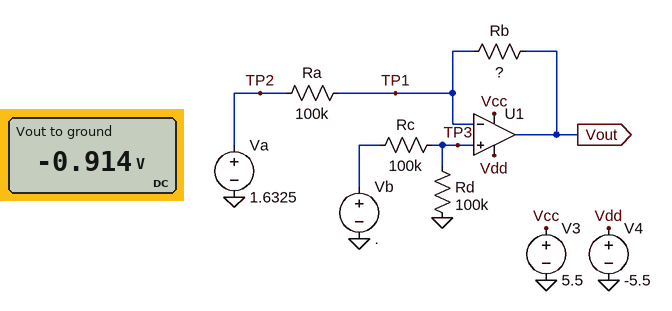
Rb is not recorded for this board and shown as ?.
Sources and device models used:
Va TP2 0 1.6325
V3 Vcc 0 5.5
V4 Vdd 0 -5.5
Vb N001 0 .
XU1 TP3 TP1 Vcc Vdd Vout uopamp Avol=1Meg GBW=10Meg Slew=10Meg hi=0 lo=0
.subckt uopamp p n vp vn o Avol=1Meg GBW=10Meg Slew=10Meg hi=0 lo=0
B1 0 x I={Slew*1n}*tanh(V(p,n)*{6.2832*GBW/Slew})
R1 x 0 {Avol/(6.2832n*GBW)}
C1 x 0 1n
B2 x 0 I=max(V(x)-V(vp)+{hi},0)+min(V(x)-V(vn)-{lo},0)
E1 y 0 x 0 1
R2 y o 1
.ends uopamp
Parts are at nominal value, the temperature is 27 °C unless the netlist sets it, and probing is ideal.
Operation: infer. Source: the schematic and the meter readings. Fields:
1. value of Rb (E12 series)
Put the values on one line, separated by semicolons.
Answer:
56 kΩ
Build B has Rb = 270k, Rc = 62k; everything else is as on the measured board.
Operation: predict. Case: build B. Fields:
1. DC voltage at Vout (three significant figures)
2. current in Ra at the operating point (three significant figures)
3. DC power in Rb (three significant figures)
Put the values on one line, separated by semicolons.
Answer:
-4.41 V; 16.3 µA; 72.0 µW
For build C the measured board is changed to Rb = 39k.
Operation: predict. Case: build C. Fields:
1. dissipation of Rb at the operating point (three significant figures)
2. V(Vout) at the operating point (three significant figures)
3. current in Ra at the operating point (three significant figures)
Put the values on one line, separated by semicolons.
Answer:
10.4 µW; -637 mV; 16.3 µA
